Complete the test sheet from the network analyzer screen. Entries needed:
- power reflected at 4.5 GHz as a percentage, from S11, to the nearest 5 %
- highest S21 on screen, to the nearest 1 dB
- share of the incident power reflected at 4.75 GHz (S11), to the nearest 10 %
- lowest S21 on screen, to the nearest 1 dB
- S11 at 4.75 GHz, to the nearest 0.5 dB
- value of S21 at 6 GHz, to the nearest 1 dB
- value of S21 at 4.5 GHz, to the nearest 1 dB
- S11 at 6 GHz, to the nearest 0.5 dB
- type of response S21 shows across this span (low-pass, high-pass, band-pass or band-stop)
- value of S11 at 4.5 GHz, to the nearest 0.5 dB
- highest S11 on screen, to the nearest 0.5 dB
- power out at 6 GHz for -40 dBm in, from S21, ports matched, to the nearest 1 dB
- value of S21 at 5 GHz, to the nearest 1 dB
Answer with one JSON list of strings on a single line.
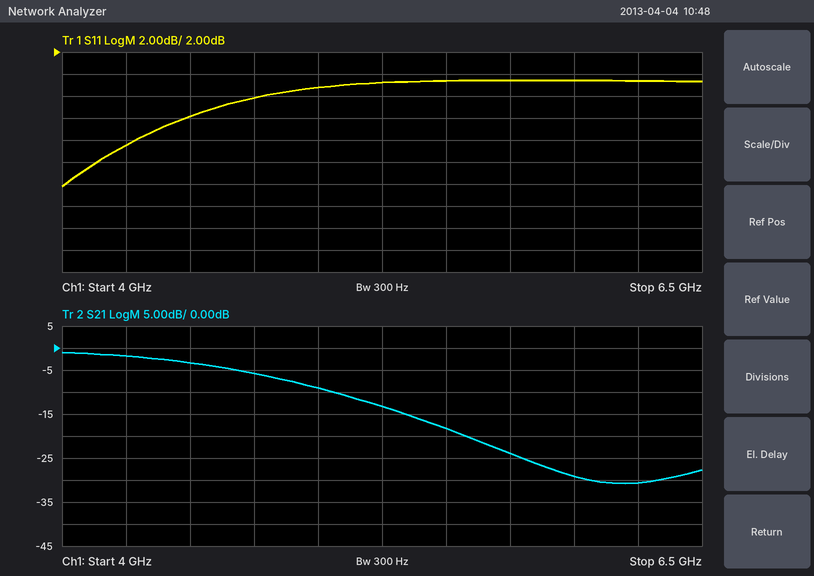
["40 %", "-1 dB", "60 %", "-31 dB", "-2.0 dB", "-29 dB", "-3 dB", "-0.5 dB", "low-pass", "-4.0 dB", "-0.5 dB", "-69 dBm", "-9 dB"]
